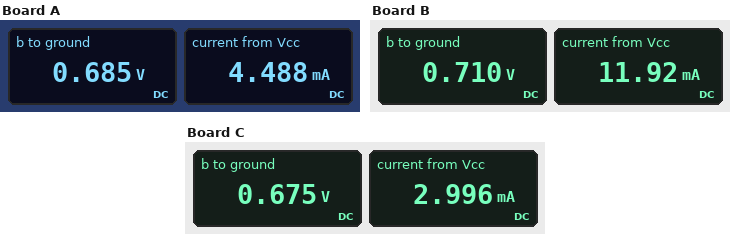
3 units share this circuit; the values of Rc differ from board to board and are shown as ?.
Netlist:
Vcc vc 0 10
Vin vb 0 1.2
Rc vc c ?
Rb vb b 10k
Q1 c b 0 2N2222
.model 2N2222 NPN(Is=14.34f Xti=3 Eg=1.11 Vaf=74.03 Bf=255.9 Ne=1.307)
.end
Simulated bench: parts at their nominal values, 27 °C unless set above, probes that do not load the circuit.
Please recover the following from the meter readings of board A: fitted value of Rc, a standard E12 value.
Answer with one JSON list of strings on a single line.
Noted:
["2.2 kΩ"]
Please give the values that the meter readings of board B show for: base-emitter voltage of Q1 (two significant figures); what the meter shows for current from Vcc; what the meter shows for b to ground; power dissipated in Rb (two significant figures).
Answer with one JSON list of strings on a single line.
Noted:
["710 mV", "11.92 mA", "0.710 V", "24 µW"]
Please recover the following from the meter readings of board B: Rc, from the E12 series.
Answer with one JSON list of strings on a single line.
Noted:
["820 Ω"]
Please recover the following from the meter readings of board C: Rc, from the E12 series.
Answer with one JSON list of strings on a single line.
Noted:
["3.3 kΩ"]
